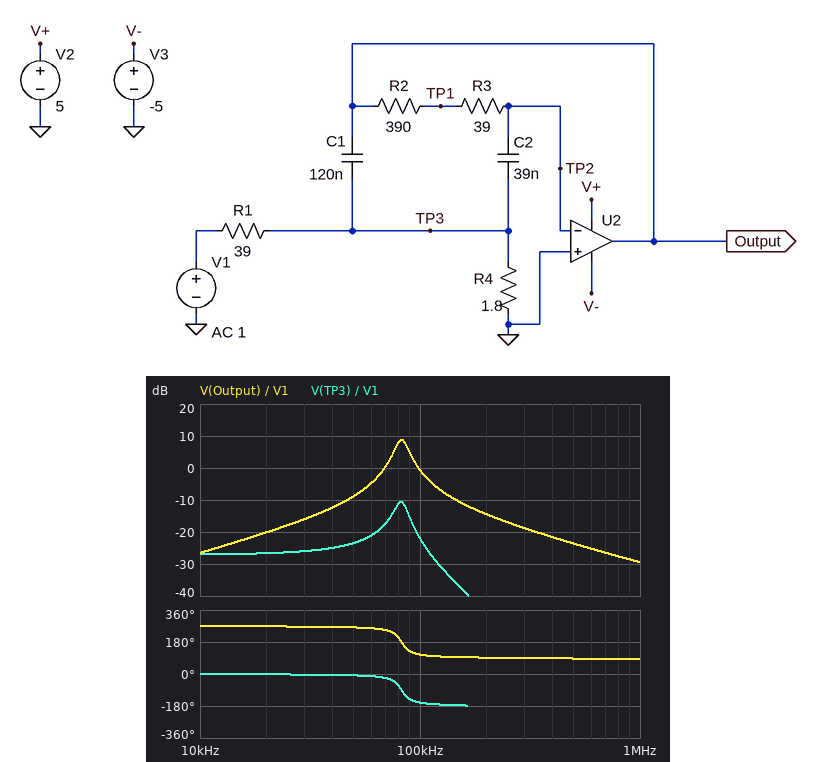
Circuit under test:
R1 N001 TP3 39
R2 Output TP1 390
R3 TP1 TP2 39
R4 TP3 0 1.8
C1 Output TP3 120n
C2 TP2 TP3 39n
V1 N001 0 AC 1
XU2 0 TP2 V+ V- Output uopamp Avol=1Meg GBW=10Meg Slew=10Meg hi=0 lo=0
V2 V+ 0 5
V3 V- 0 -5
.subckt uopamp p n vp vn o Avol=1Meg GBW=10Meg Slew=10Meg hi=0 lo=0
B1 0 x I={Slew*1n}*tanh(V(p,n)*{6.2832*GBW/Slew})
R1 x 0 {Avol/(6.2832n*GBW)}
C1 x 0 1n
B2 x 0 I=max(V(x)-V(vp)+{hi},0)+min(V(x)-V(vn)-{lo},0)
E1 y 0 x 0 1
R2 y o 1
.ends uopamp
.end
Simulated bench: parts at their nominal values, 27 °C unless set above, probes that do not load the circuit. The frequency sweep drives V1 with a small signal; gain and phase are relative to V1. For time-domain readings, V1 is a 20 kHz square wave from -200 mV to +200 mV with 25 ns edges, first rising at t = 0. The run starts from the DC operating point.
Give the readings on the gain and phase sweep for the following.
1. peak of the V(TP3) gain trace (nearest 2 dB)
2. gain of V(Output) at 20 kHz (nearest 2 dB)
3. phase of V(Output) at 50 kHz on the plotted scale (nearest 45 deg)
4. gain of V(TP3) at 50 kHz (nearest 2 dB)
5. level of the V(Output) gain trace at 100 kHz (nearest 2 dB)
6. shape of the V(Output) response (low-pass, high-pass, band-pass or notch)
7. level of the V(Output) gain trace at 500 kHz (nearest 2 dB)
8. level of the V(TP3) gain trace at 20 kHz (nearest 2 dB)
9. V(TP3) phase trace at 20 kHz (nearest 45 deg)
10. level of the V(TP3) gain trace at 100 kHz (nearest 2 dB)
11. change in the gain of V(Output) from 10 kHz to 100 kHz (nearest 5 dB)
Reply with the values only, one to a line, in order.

-10 dB
-20 dB
270 deg
-24 dB
0 dB
band-pass
-24 dB
-26 dB
0 deg
-22 dB
25 dB
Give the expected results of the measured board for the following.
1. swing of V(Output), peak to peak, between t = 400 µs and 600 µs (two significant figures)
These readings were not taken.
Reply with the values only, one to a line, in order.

200 mV
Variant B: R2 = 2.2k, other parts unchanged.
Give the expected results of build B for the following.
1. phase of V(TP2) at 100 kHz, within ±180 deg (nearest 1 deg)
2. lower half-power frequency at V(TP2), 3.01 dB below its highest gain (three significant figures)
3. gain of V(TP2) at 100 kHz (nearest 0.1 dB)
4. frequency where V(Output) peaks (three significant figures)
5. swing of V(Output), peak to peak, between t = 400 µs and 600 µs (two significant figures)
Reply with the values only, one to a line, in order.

5 deg
35.1 kHz
-48.8 dB
36.1 kHz
390 mV
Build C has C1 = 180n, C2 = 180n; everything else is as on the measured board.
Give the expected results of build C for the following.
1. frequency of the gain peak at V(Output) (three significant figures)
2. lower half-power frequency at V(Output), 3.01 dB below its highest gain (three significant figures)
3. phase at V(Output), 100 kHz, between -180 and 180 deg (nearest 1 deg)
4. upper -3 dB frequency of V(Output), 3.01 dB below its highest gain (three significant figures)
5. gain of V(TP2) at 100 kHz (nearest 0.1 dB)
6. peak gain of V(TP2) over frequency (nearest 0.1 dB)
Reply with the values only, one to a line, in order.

31.7 kHz
29.9 kHz
92 deg
33.7 kHz
-52.3 dB
-35.0 dB
